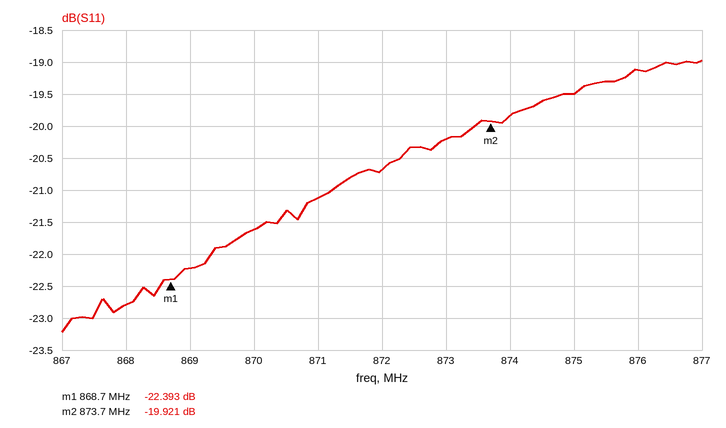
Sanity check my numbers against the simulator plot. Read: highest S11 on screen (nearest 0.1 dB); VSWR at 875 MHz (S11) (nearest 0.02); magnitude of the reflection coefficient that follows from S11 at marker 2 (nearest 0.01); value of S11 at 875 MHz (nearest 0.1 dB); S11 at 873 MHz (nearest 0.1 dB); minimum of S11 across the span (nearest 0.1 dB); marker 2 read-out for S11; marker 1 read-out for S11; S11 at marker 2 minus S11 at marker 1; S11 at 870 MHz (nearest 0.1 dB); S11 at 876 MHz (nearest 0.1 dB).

-19.0 dB
1.24
0.10
-19.5 dB
-20.2 dB
-23.2 dB
-19.921 dB
-22.393 dB
2.472 dB
-21.6 dB
-19.1 dB
